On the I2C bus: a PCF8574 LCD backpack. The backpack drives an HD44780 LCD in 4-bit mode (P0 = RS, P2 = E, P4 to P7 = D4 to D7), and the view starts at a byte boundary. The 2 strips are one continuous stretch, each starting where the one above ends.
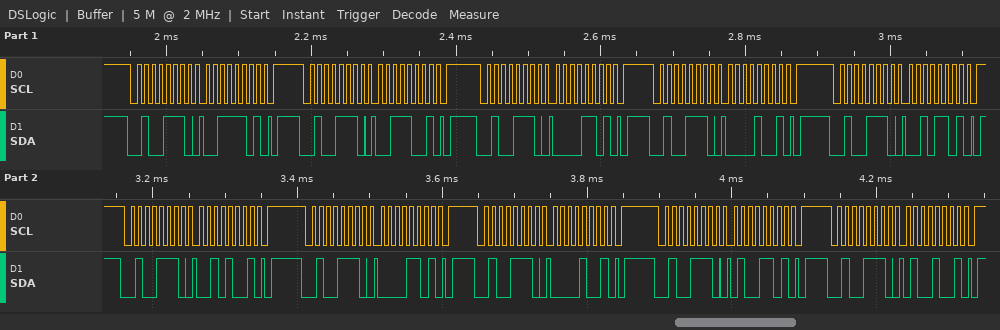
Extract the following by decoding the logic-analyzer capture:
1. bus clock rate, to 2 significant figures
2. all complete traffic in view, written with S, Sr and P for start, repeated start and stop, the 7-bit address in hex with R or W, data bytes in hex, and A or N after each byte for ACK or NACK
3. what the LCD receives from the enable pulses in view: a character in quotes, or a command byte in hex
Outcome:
100 kHz
S 27W A 3D A P S 27W A 39 A P S 27W A 0D A P S 27W A 09 A P S 27W A 2D A P S 27W A 29 A P S 27W A 0D A P S 27W A 09 A P S 27W A 4D A P S 27W A 49 A P
'0' ' '
